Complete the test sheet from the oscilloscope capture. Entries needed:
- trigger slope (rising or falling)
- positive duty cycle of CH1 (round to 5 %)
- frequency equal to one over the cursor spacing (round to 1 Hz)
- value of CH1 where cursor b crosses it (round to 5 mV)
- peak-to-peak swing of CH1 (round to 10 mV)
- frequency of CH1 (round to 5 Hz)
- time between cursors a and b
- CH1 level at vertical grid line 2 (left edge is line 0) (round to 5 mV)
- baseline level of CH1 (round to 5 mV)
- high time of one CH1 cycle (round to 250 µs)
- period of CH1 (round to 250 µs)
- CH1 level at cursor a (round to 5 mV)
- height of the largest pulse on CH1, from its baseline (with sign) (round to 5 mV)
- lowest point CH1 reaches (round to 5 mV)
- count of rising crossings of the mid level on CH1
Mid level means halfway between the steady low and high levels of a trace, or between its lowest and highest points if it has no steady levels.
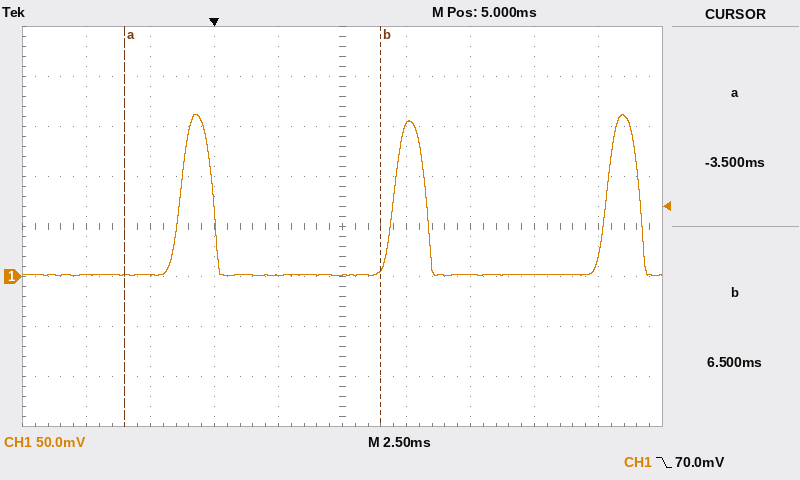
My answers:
falling
15 %
100 Hz
10 mV
160 mV
120 Hz
10.00 ms
0 mV
0 mV
1.25 ms
8.25 ms
0 mV
+160 mV
0 mV
3
